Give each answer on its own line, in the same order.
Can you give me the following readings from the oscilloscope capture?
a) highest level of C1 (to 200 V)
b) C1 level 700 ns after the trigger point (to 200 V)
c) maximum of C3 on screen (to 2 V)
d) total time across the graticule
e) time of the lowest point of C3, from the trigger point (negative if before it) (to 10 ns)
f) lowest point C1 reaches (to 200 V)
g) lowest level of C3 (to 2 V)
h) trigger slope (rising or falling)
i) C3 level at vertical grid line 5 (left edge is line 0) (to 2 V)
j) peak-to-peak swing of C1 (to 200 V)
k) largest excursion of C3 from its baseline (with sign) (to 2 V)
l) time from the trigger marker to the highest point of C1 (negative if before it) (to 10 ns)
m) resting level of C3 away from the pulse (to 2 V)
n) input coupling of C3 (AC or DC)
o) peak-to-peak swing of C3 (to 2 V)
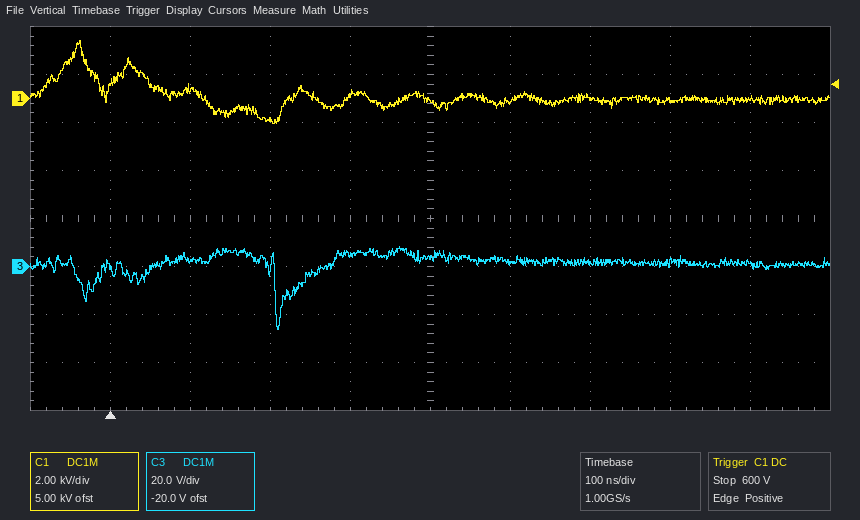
2.4 kV
0.0 kV
8 V
1 µs
+210 ns
-1.0 kV
-26 V
rising
4 V
3.4 kV
-28 V
-40 ns
2 V
DC
34 V
